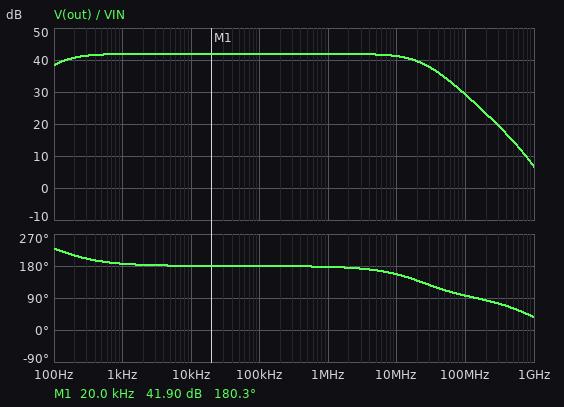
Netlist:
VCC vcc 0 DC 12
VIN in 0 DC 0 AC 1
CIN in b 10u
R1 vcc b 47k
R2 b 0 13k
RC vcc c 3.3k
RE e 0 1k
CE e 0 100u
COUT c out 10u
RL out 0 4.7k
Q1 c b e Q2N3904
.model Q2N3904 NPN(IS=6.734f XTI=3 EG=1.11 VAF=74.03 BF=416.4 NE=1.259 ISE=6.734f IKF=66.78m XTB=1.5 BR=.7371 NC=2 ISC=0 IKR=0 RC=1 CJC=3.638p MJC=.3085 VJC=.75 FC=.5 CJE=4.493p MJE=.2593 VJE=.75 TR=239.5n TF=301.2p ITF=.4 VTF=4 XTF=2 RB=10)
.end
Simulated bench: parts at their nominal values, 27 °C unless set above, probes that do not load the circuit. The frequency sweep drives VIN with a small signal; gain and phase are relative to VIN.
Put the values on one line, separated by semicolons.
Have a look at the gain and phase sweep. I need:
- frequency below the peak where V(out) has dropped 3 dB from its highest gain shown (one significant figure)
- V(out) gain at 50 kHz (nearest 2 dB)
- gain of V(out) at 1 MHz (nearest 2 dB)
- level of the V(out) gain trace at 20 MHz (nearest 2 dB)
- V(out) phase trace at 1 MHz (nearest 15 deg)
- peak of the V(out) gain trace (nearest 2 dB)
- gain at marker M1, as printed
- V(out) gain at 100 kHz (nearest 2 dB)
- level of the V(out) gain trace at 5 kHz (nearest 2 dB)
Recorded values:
100 Hz; 42 dB; 42 dB; 40 dB; 180 deg; 42 dB; 41.90 dB; 42 dB; 42 dB
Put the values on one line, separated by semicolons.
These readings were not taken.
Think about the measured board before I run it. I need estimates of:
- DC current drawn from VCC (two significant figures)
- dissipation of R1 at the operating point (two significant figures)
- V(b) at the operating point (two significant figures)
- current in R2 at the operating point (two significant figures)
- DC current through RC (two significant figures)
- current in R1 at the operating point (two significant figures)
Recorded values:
2.0 mA; 1.9 mW; 2.5 V; 190 µA; 1.8 mA; 200 µA
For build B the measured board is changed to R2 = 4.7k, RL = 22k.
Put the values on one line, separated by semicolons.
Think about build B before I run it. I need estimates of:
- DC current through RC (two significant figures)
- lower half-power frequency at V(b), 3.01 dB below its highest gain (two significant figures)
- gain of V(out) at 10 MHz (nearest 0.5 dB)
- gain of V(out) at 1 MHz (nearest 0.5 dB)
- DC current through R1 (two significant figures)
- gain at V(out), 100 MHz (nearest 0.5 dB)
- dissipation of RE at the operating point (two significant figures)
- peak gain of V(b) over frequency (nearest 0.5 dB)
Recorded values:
430 µA; 4.1 Hz; 33.0 dB; 33.5 dB; 230 µA; 22.5 dB; 190 µW; 0 dB
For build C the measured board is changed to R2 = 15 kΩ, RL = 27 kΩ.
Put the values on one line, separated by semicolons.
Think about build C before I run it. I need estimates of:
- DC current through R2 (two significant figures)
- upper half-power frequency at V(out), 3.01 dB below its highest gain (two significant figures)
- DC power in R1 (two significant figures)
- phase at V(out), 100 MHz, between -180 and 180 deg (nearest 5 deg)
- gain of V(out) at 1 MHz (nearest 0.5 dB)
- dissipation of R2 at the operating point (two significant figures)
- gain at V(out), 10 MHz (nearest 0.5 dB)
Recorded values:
180 µA; 14 MHz; 1.8 mW; 90 deg; 46.5 dB; 500 µW; 44.5 dB
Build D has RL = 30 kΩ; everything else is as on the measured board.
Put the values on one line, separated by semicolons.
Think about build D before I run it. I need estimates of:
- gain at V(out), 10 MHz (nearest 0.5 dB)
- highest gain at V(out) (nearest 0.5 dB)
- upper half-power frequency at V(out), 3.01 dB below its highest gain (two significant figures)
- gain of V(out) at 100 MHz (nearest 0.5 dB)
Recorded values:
44.0 dB; 45.5 dB; 16 MHz; 29.5 dB
